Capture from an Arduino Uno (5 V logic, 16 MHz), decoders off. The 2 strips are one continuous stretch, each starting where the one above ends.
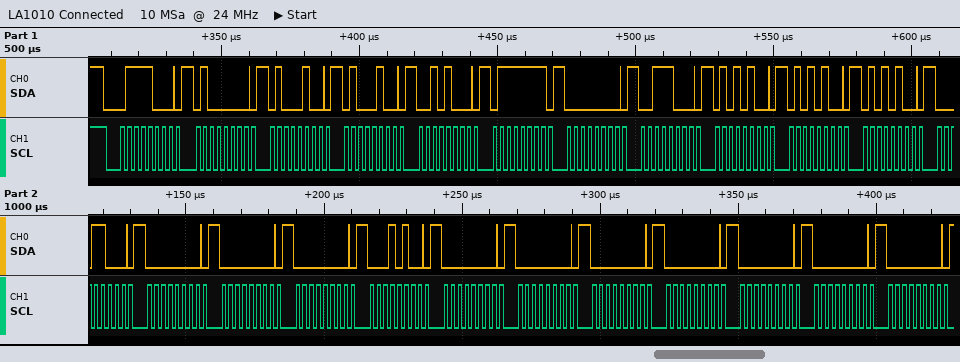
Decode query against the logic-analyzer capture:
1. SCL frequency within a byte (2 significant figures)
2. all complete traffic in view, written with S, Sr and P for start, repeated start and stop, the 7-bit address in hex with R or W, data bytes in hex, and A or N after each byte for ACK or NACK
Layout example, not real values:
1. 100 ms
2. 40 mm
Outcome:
1. 400 kHz
2. S 3CW A 40 A 44 A 44 A 28 A 7F A 00 A 38 A 54 A 54 A 54 A 18 A 00 A 00 A 00 A 14 A 00 A 00 A 00 A 00 A 00 A 00 A 00 A
